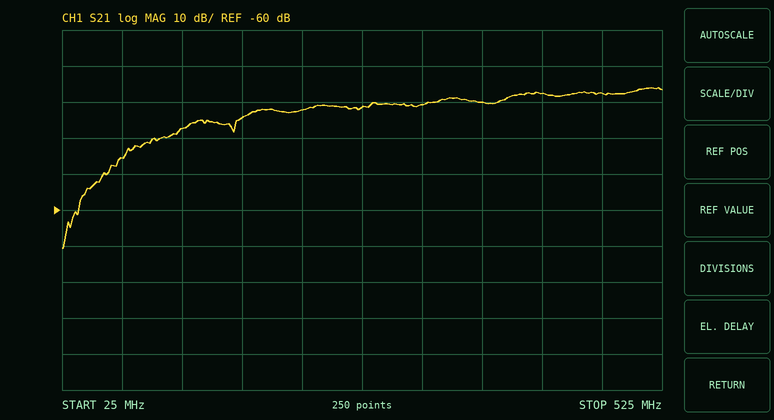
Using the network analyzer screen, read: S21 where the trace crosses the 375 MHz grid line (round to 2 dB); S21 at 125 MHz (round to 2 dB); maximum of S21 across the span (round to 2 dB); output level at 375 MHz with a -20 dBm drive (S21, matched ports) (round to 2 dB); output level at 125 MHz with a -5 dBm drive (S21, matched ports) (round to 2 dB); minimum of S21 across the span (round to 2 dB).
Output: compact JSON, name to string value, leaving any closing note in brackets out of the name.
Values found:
{"S21 where the trace crosses the 375 MHz grid line": "-30 dB", "S21 at 125 MHz": "-38 dB", "maximum of S21 across the span": "-26 dB", "output level at 375 MHz with a -20 dBm drive (S21, matched ports)": "-50 dBm", "output level at 125 MHz with a -5 dBm drive (S21, matched ports)": "-42 dBm", "minimum of S21 across the span": "-70 dB"}
